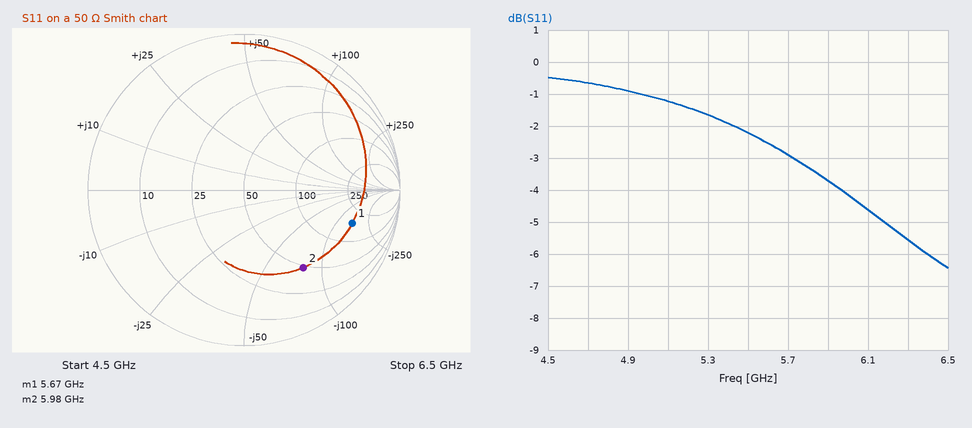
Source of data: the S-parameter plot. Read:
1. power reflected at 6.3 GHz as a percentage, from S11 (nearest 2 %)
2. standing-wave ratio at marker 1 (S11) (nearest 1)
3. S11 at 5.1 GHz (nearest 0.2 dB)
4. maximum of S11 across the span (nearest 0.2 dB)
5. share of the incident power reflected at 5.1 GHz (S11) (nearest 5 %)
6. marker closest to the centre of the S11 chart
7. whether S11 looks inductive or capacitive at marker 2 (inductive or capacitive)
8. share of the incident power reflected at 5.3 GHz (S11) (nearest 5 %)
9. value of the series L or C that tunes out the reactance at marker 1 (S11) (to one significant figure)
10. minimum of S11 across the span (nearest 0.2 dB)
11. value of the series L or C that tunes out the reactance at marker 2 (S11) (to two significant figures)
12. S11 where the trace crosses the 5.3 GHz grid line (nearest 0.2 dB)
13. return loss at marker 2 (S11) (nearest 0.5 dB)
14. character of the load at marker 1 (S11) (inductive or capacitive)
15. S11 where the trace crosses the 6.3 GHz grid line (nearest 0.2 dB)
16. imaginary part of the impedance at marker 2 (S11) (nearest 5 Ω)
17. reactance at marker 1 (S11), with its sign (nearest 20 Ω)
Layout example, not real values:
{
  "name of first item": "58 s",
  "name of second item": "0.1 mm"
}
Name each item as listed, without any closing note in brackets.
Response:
{
  "power reflected at 6.3 GHz as a percentage, from S11": "28 %",
  "standing-wave ratio at marker 1 (S11)": "6",
  "S11 at 5.1 GHz": "-1.2 dB",
  "maximum of S11 across the span": "-0.4 dB",
  "share of the incident power reflected at 5.1 GHz (S11)": "75 %",
  "marker closest to the centre of the S11 chart": "marker 2",
  "whether S11 looks inductive or capacitive at marker 2": "capacitive",
  "share of the incident power reflected at 5.3 GHz (S11)": "70 %",
  "value of the series L or C that tunes out the reactance at marker 1 (S11)": "4 nH",
  "minimum of S11 across the span": "-6.4 dB",
  "value of the series L or C that tunes out the reactance at marker 2 (S11)": "2.1 nH",
  "S11 where the trace crosses the 5.3 GHz grid line": "-1.6 dB",
  "return loss at marker 2 (S11)": "4.0 dB",
  "character of the load at marker 1 (S11)": "capacitive",
  "S11 where the trace crosses the 6.3 GHz grid line": "-5.6 dB",
  "imaginary part of the impedance at marker 2 (S11)": "-80 Ω",
  "reactance at marker 1 (S11), with its sign": "-160 Ω"
}
